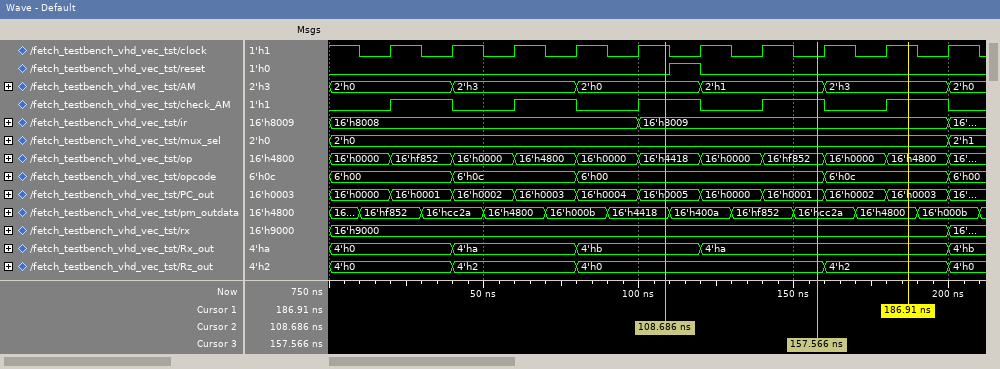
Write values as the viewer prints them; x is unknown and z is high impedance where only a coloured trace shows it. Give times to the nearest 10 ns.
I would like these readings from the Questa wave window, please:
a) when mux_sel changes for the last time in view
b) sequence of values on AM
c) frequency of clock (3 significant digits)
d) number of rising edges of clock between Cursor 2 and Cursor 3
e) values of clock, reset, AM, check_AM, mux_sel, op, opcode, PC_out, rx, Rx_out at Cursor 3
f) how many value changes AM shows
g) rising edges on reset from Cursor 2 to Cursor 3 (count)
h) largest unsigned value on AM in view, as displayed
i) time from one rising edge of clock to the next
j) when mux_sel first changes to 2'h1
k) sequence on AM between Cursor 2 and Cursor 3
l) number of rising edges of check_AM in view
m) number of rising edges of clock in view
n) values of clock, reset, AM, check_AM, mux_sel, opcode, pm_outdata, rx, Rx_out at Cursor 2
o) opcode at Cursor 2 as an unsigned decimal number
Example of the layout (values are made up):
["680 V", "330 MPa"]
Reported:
["200 ns", "2'h0, 2'h3, 2'h0, 2'h1, 2'h3, 2'h0", "50.0 MHz", "2", "clock=0, reset=0, AM=2'h1, check_AM=1, mux_sel=2'h0, op=16'hf852, opcode=6'h00, PC_out=16'h0001, rx=16'h9000, Rx_out=4'ha", "5", "1", "2'h3", "20 ns", "200 ns", "2'h0, 2'h1", "5", "10", "clock=1, reset=0, AM=2'h0, check_AM=1, mux_sel=2'h0, opcode=6'h00, pm_outdata=16'h4418, rx=16'h9000, Rx_out=4'hb", "0"]
